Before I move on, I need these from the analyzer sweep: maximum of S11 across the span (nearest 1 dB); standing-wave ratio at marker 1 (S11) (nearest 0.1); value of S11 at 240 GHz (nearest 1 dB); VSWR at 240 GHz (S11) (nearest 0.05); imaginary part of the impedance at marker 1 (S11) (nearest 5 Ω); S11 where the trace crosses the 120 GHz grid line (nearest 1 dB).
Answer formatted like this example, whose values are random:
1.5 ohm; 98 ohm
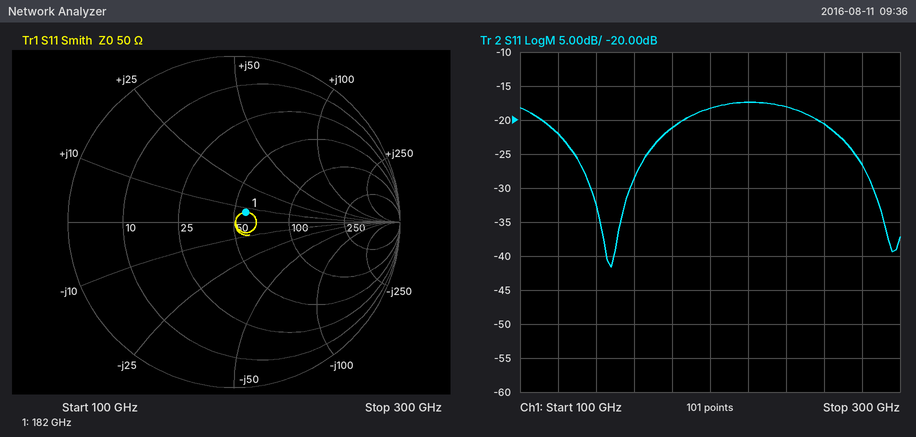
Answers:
-17 dB; 1.2; -18 dB; 1.30; +5 Ω; -22 dB
